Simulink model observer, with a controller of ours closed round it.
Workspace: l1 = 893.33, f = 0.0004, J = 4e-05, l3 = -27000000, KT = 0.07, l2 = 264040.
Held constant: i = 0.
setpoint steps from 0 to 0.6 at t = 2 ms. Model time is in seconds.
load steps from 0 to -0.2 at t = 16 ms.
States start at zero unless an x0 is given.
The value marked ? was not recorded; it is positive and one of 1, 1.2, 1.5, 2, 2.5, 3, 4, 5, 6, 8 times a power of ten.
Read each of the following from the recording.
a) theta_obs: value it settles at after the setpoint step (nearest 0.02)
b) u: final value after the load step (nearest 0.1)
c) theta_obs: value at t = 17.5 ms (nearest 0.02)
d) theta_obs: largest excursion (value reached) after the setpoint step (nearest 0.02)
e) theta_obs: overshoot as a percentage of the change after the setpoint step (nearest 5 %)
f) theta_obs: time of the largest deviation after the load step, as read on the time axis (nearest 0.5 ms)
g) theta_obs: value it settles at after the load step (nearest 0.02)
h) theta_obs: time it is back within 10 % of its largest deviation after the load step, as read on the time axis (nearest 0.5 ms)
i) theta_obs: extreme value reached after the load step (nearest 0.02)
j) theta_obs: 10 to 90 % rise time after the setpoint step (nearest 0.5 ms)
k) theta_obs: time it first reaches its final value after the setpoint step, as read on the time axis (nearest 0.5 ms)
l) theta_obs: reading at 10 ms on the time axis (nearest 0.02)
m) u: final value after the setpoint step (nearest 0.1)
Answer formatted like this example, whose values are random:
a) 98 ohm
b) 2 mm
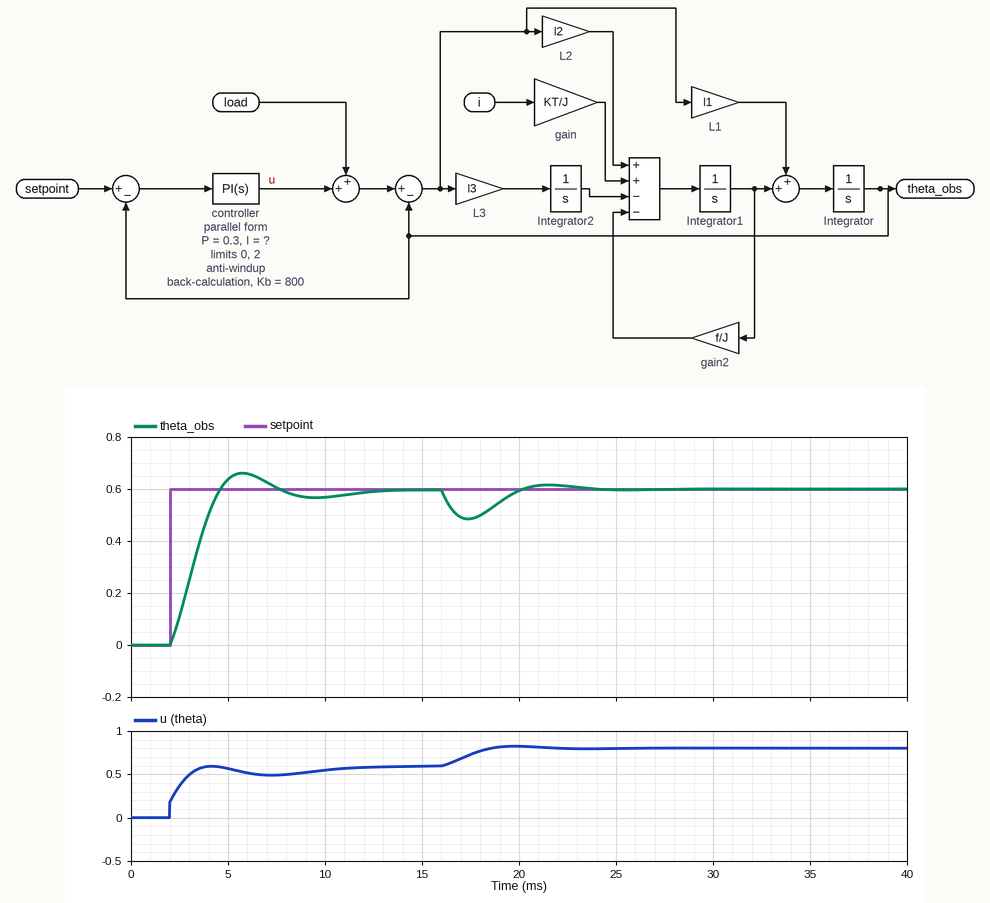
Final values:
a) 0.60
b) 0.8
c) 0.48
d) 0.66
e) 10 %
f) 17.5 ms
g) 0.60
h) 22.5 ms
i) 0.48
j) 2.0 ms
k) 4.5 ms
l) 0.56
m) 0.6
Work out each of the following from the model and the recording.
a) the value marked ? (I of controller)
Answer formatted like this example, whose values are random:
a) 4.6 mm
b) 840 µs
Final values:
a) 800
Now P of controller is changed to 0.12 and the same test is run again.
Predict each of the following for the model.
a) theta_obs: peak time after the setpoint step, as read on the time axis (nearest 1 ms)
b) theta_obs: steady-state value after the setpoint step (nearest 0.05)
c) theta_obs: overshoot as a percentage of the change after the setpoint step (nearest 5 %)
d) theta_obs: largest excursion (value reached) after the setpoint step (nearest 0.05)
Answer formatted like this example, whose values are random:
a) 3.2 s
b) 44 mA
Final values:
a) 6 ms
b) 0.60
c) 15 %
d) 0.70
